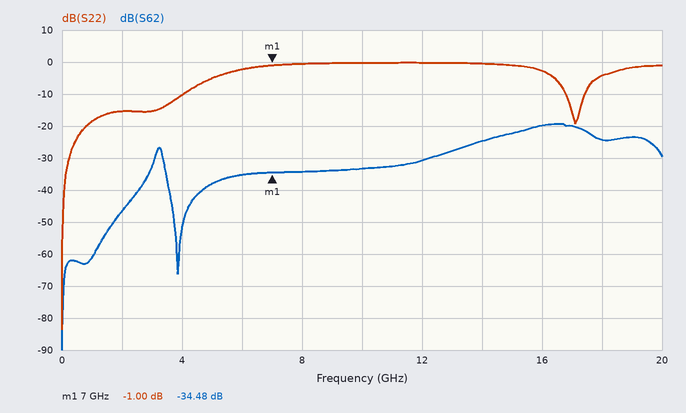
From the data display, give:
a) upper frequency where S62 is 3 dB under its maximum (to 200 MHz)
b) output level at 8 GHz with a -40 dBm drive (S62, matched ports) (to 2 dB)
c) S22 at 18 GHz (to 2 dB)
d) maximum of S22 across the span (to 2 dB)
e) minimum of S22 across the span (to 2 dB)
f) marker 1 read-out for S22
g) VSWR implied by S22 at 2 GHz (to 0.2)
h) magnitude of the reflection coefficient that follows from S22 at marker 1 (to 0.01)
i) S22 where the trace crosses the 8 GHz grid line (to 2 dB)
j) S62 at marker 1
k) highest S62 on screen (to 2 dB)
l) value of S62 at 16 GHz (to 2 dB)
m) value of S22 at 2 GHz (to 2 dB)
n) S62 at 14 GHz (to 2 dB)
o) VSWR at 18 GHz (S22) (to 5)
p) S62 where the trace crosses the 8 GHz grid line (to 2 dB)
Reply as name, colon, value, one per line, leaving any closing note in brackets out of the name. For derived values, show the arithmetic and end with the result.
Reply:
upper frequency where S62 is 3 dB under its maximum: 17.6 GHz
output level at 8 GHz with a -40 dBm drive (S62, matched ports): -40 dBm + (-34 dB) = -74 dBm
S22 at 18 GHz: -4 dB
maximum of S22 across the span: 0 dB
minimum of S22 across the span: -84 dB
marker 1 read-out for S22: -1.00 dB
VSWR implied by S22 at 2 GHz: |Γ| = 10^(-16/20) = 0.1585; VSWR = (1 + 0.1585)/(1 − 0.1585) ≈ 1.4
magnitude of the reflection coefficient that follows from S22 at marker 1: 10^(-1/20) ≈ 0.89
S22 where the trace crosses the 8 GHz grid line: 0 dB
S62 at marker 1: -34.48 dB
highest S62 on screen: -20 dB
value of S62 at 16 GHz: -20 dB
value of S22 at 2 GHz: -16 dB
S62 at 14 GHz: -24 dB
VSWR at 18 GHz (S22): |Γ| = 10^(-4/20) = 0.6310; VSWR = (1 + 0.6310)/(1 − 0.6310) ≈ 4.42, so 5 to the nearest 5
S62 where the trace crosses the 8 GHz grid line: -34 dB
